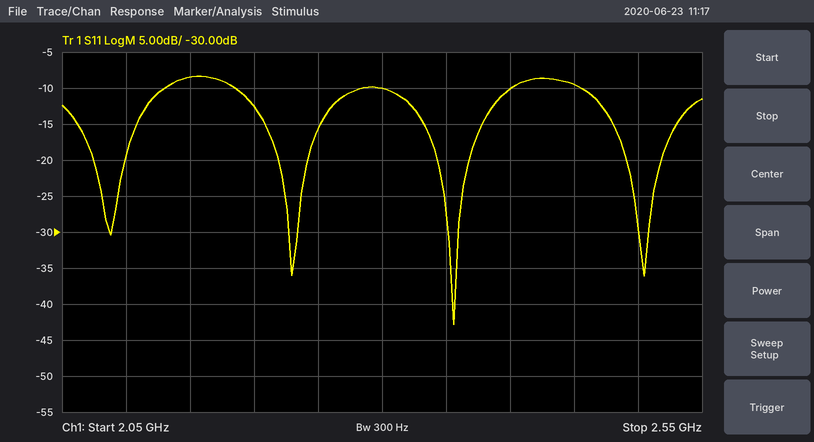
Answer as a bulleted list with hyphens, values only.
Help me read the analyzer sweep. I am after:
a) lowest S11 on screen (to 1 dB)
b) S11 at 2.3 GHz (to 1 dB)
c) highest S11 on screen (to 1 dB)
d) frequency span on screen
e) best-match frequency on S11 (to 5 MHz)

- -43 dB
- -10 dB
- -8 dB
- 500 MHz
- 2.355 GHz
